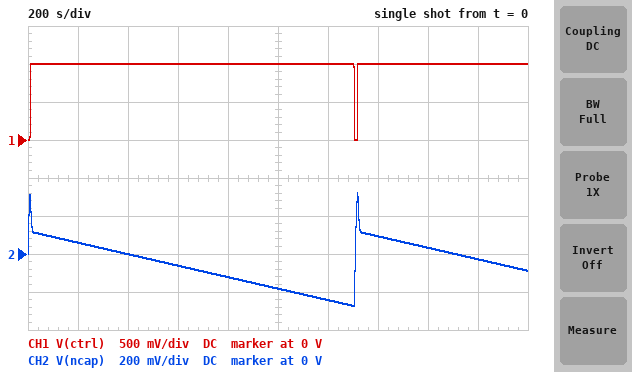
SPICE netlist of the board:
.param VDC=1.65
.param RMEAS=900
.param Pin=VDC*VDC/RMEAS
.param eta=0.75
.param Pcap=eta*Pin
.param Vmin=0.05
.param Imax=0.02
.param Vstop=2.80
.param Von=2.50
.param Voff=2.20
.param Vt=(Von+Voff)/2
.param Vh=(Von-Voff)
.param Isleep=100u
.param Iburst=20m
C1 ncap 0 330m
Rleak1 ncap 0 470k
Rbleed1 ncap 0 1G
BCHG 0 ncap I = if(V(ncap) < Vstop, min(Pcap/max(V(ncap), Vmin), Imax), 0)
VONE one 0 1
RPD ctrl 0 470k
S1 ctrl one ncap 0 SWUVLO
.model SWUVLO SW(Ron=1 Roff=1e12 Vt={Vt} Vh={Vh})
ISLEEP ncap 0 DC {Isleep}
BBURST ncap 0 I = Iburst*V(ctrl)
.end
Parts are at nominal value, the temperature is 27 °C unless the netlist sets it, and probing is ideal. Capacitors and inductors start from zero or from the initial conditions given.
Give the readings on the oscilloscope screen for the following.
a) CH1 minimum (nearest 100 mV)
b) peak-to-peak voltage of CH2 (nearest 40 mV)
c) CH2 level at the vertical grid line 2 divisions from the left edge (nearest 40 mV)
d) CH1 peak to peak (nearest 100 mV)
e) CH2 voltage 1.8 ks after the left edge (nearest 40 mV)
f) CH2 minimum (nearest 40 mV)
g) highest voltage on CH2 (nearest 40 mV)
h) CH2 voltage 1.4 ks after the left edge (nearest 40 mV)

0 V
600 mV
0 V
1.0 V
-40 mV
-280 mV
320 mV
80 mV
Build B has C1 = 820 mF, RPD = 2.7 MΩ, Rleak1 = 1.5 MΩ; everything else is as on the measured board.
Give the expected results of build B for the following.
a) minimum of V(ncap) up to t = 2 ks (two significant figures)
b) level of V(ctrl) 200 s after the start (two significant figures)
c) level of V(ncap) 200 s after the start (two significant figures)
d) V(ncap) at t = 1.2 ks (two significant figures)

-120 mV
1.0 V
96 mV
-26 mV
